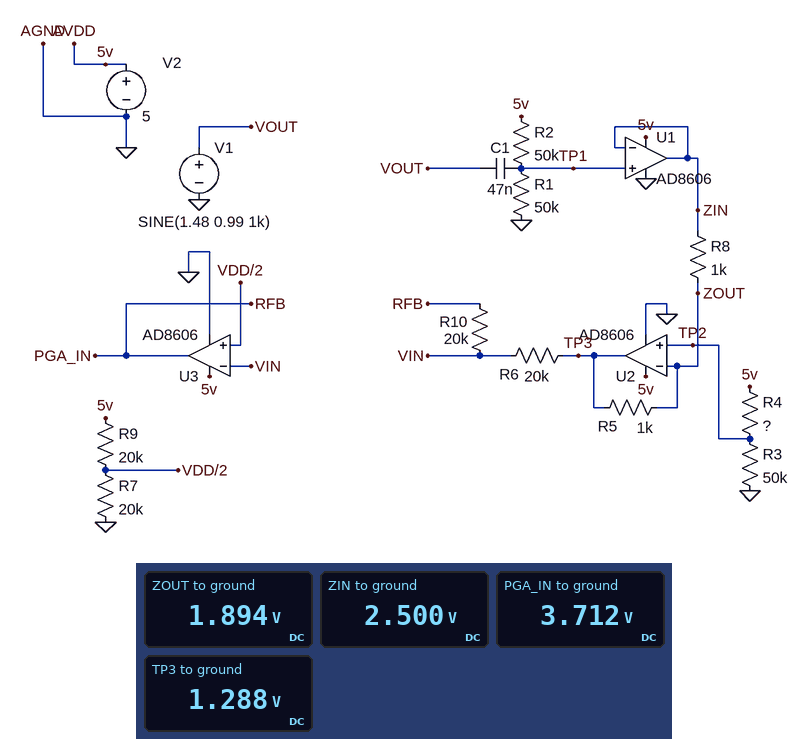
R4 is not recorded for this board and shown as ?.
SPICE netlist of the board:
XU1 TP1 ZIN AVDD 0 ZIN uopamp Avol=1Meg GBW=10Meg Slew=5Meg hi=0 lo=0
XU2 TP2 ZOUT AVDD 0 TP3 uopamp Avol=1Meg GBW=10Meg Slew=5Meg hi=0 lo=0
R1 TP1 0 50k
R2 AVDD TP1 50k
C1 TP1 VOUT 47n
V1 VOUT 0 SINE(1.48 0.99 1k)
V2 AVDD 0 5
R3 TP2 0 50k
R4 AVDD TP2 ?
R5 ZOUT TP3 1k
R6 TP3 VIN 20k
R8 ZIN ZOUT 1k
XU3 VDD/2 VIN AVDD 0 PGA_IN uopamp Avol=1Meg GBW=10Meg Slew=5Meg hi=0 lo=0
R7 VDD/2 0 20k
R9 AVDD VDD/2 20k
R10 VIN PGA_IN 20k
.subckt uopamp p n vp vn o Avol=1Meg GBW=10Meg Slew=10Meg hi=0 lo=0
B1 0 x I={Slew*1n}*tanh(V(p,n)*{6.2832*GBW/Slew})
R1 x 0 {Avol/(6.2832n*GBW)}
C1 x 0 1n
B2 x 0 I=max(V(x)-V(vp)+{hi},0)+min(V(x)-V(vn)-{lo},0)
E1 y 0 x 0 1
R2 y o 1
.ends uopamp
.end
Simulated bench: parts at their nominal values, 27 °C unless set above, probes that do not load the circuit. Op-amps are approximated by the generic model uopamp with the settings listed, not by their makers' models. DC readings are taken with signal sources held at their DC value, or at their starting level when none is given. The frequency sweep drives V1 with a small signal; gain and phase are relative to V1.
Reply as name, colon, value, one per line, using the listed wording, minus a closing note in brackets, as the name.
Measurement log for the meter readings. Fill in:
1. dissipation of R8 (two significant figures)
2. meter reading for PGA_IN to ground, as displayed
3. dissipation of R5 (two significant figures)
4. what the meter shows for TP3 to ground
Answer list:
dissipation of R8: 370 µW
meter reading for PGA_IN to ground, as displayed: 3.712 V
dissipation of R5: 370 µW
what the meter shows for TP3 to ground: 1.288 V
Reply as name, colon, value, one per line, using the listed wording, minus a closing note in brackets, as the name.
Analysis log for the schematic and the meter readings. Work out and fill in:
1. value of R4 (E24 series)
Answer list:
value of R4: 82 kΩ
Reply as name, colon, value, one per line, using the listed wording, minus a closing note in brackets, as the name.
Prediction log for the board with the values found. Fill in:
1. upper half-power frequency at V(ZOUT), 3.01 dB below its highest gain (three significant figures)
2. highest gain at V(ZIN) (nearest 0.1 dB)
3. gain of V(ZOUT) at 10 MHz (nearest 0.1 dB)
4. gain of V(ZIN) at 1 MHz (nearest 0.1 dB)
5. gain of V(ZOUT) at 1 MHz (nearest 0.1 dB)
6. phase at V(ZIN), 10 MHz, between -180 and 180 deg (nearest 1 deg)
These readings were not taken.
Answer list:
upper half-power frequency at V(ZOUT), 3.01 dB below its highest gain: 17.8 MHz
highest gain at V(ZIN): 0 dB
gain of V(ZOUT) at 10 MHz: -10.0 dB
gain of V(ZIN) at 1 MHz: 0 dB
gain of V(ZOUT) at 1 MHz: -20.2 dB
phase at V(ZIN), 10 MHz, between -180 and 180 deg: -45 deg
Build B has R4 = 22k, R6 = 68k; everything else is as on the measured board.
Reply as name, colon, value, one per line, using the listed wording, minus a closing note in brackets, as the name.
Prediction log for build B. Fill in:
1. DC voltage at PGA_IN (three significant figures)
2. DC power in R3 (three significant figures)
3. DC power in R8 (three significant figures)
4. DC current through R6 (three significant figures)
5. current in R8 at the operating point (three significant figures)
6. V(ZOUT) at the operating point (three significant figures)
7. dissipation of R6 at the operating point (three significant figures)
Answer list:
DC voltage at PGA_IN: 1.93 V
DC power in R3: 241 µW
DC power in R8: 945 µW
DC current through R6: 28.6 µA
current in R8 at the operating point: 972 µA
V(ZOUT) at the operating point: 3.47 V
dissipation of R6 at the operating point: 55.6 µW
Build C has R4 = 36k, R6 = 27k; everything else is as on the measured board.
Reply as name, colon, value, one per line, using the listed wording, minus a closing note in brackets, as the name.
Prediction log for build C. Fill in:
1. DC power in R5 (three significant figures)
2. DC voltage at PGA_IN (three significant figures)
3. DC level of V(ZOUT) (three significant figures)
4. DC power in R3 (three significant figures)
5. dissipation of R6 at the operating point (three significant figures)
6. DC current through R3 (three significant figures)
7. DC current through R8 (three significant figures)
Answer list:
DC power in R5: 166 µW
DC voltage at PGA_IN: 1.90 V
DC level of V(ZOUT): 2.91 V
DC power in R3: 169 µW
dissipation of R6 at the operating point: 24.5 µW
DC current through R3: 58.1 µA
DC current through R8: 407 µA
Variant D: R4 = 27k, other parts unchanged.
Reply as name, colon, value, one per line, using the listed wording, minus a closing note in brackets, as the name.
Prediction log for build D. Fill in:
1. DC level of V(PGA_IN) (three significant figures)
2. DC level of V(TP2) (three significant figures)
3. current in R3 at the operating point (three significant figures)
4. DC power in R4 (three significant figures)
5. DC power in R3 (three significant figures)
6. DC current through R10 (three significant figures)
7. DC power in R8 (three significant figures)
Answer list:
DC level of V(PGA_IN): 1.01 V
DC level of V(TP2): 3.25 V
current in R3 at the operating point: 64.9 µA
DC power in R4: 114 µW
DC power in R3: 211 µW
DC current through R10: 74.7 µA
DC power in R8: 558 µW
